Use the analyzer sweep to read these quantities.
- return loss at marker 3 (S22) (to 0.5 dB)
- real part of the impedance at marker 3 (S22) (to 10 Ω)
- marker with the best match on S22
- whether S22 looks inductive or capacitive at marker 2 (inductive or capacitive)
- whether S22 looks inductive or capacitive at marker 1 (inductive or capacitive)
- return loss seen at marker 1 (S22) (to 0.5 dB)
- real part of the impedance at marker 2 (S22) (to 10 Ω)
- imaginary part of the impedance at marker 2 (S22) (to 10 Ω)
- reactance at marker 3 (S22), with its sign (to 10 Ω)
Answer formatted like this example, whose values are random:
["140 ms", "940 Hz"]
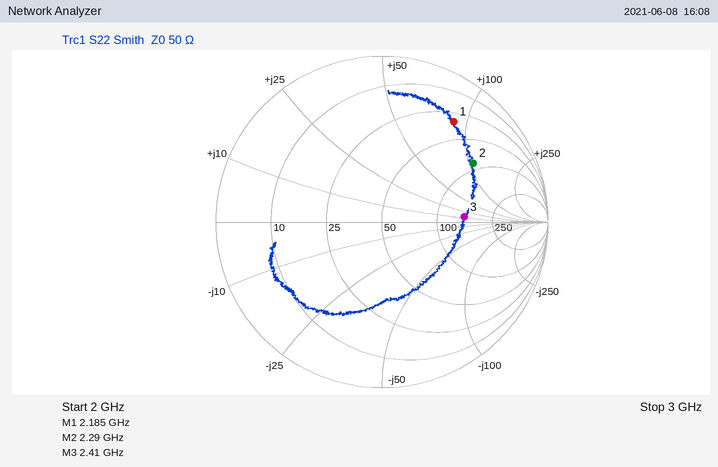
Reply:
["6.0 dB", "150 Ω", "marker 3", "inductive", "inductive", "2.5 dB", "90 Ω", "+110 Ω", "+10 Ω"]
